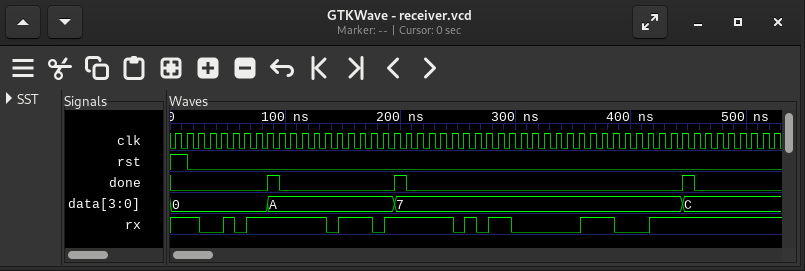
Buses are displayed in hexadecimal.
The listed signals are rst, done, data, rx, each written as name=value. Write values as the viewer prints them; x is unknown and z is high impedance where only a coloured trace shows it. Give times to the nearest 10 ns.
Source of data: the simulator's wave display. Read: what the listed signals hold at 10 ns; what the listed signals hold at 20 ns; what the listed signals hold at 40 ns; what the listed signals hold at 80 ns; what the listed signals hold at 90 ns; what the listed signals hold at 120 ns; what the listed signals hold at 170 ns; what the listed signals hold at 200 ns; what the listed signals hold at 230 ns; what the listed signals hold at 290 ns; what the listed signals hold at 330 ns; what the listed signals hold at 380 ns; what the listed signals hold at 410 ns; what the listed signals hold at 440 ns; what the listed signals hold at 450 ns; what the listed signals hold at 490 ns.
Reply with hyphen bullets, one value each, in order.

- rst=1, done=0, data=0, rx=1
- rst=0, done=0, data=0, rx=1
- rst=0, done=0, data=0, rx=0
- rst=0, done=0, data=0, rx=1
- rst=0, done=1, data=A, rx=1
- rst=0, done=0, data=A, rx=1
- rst=0, done=0, data=A, rx=1
- rst=0, done=1, data=7, rx=1
- rst=0, done=0, data=7, rx=1
- rst=0, done=0, data=7, rx=1
- rst=0, done=0, data=7, rx=0
- rst=0, done=0, data=7, rx=1
- rst=0, done=0, data=7, rx=0
- rst=0, done=0, data=7, rx=1
- rst=0, done=1, data=C, rx=1
- rst=0, done=0, data=C, rx=1
